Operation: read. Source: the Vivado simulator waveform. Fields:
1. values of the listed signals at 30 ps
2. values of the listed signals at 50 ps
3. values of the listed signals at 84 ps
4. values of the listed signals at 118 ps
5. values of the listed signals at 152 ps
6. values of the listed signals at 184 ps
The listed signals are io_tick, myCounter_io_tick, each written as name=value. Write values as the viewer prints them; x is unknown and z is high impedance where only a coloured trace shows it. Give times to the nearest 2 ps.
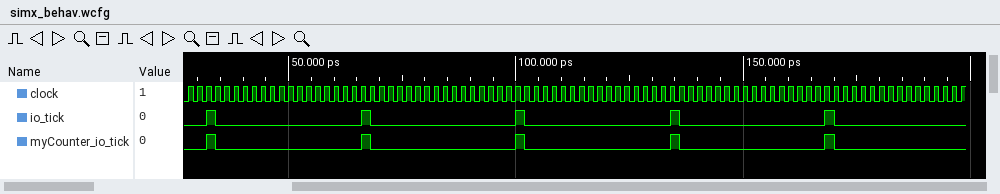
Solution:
io_tick=0, myCounter_io_tick=0
io_tick=0, myCounter_io_tick=0
io_tick=0, myCounter_io_tick=0
io_tick=0, myCounter_io_tick=0
io_tick=0, myCounter_io_tick=0
io_tick=0, myCounter_io_tick=0
